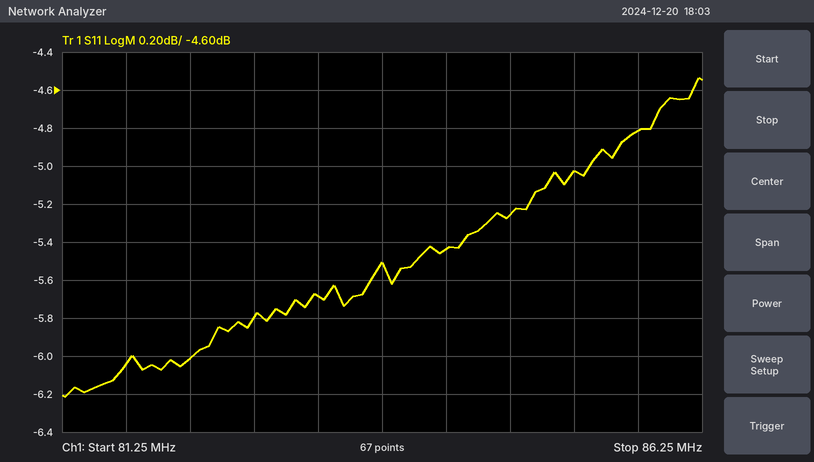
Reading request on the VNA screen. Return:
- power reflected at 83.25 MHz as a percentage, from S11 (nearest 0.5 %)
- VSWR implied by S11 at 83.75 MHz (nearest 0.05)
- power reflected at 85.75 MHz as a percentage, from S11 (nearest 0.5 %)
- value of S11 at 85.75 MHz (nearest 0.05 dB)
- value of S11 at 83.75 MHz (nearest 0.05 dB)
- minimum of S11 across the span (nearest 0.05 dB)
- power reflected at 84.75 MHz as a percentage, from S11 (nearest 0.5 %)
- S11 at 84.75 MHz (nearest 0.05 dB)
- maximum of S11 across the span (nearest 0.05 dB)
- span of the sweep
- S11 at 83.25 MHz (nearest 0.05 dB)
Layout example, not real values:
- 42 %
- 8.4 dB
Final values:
- 27.0 %
- 3.25
- 33.0 %
- -4.80 dB
- -5.50 dB
- -6.20 dB
- 30.0 %
- -5.25 dB
- -4.55 dB
- 5 MHz
- -5.70 dB
